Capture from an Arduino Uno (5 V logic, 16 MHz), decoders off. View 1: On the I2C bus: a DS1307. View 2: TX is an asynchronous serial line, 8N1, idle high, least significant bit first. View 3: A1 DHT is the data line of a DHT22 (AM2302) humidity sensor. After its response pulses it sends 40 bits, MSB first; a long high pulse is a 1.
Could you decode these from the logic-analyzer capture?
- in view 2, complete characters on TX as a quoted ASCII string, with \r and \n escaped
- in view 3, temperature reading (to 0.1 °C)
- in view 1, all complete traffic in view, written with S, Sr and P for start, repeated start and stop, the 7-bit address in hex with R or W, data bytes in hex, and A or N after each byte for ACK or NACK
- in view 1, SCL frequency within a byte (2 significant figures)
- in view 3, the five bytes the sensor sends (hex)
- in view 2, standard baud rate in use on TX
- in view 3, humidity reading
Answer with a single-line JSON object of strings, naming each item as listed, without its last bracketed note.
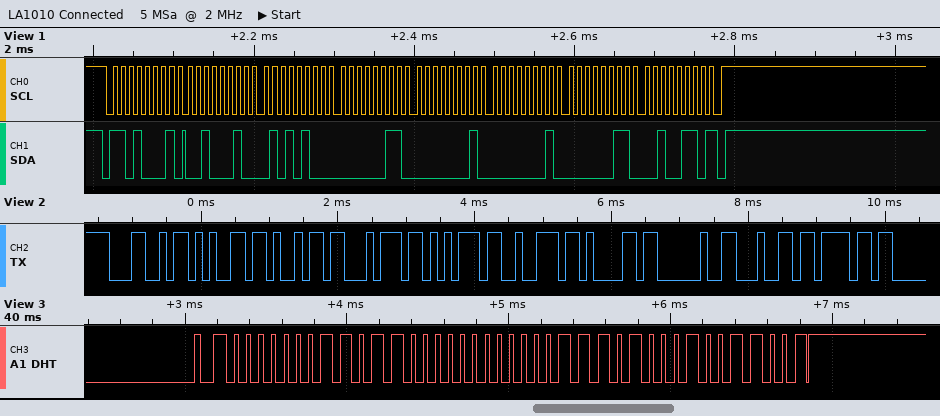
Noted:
{"in view 2, complete characters on TX as a quoted ASCII string, with \\r and \\n escaped": "\"Leitura do\"", "in view 3, temperature reading": "23.2 °C", "in view 1, all complete traffic in view, written with S, Sr and P for start, repeated start and stop, the 7-bit address in hex with R or W, data bytes in hex, and A or N after each byte for ACK or NACK": "S 68R A 22 A 54 A 03 A 01 A 01 A 03 A 26 N P", "in view 1, SCL frequency within a byte": "100 kHz", "in view 3, the five bytes the sensor sends": "01 B0 00 E8 99", "in view 2, standard baud rate in use on TX": "9600 baud", "in view 3, humidity reading": "43.2 %"}
